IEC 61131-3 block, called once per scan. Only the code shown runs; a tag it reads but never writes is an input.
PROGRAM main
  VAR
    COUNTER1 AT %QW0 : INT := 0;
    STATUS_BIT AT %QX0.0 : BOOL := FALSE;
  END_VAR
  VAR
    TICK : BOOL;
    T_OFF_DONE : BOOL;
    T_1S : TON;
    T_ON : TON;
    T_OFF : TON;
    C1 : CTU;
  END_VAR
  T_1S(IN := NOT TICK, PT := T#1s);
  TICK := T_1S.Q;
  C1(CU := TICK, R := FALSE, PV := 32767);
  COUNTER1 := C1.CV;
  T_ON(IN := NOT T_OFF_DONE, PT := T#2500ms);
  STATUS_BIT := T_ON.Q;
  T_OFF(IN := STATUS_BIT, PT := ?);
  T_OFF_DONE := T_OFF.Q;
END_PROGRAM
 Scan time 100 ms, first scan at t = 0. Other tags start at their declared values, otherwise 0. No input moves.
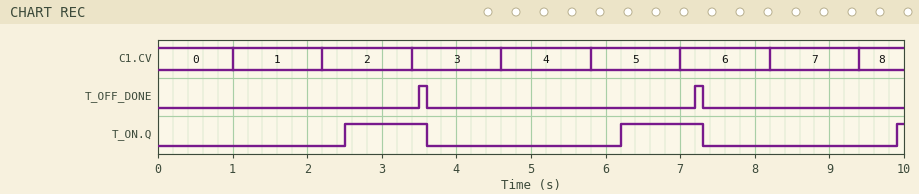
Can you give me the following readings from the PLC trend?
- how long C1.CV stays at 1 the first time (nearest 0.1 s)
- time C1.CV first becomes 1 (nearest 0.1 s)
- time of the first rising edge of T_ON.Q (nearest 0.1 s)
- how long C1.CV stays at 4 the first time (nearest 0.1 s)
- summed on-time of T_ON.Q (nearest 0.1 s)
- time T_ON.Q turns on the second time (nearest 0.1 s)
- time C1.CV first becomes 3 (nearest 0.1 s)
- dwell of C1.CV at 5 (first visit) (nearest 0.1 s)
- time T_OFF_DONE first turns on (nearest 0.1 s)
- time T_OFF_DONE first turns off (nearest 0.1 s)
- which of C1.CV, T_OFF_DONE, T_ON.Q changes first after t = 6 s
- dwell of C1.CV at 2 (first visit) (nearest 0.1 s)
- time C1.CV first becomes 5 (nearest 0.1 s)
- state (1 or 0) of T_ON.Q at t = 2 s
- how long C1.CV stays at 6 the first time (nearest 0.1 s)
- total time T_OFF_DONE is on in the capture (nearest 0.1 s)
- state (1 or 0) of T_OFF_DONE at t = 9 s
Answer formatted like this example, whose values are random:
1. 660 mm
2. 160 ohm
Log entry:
1. 1.2 s
2. 1.0 s
3. 2.5 s
4. 1.2 s
5. 2.3 s
6. 6.2 s
7. 3.4 s
8. 1.2 s
9. 3.5 s
10. 3.6 s
11. T_ON.Q
12. 1.2 s
13. 5.8 s
14. 0
15. 1.2 s
16. 0.2 s
17. 0
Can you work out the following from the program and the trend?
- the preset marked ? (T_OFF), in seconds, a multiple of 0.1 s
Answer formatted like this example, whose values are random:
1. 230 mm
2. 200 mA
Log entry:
1. 1.0 s
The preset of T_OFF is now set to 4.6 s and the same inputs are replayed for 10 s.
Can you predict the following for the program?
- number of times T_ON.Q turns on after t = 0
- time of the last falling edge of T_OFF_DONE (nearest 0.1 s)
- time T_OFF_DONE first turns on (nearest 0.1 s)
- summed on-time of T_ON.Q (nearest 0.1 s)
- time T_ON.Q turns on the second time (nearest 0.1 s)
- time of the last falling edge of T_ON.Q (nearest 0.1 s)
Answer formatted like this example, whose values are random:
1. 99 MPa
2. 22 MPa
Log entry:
1. 2
2. 7.2 s
3. 7.1 s
4. 4.9 s
5. 9.8 s
6. 7.2 s
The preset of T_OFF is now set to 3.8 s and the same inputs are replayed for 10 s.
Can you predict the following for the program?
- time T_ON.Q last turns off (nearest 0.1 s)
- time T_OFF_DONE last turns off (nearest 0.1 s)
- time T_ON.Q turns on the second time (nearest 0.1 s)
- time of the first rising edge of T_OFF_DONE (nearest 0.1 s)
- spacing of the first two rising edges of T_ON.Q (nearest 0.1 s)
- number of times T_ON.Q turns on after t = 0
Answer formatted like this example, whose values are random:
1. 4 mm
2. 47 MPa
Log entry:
1. 6.4 s
2. 6.4 s
3. 9.0 s
4. 6.3 s
5. 6.5 s
6. 2
